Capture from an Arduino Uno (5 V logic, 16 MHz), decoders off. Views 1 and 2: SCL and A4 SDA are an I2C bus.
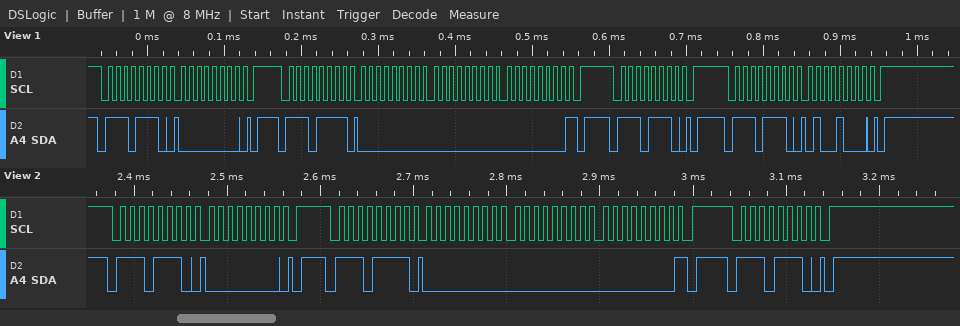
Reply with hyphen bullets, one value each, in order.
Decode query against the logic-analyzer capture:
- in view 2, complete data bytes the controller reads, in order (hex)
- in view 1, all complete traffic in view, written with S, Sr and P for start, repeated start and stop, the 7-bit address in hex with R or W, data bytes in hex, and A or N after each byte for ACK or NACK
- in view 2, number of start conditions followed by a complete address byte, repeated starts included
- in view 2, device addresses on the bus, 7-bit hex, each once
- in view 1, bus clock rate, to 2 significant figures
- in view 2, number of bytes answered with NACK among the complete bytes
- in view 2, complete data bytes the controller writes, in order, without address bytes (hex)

- 00 00 00
- S 77W A 00 A P S 77R A 00 A 00 A 00 N P S 77W A P S 77W A 48 A P
- 3
- 0x77
- 100 kHz
- 1
- 00
